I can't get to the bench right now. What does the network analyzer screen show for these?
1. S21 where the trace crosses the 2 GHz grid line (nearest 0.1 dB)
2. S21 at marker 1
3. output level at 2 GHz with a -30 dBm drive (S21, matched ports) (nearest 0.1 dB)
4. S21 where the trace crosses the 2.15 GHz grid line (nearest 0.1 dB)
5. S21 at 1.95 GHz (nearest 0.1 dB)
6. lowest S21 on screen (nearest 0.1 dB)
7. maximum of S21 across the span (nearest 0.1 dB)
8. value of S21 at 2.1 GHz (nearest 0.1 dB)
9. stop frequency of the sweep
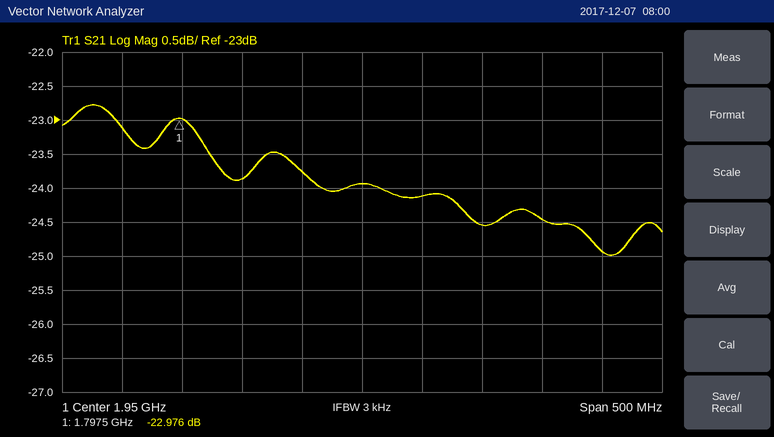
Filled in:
-24.1 dB
-22.976 dB
-54.1 dBm
-24.9 dB
-23.9 dB
-25.0 dB
-22.8 dB
-24.5 dB
2.2 GHz
